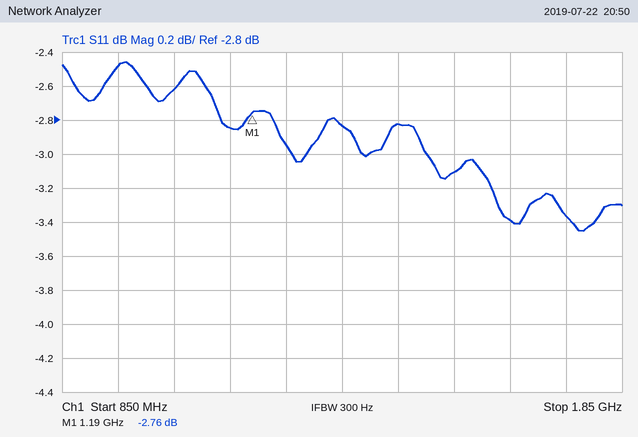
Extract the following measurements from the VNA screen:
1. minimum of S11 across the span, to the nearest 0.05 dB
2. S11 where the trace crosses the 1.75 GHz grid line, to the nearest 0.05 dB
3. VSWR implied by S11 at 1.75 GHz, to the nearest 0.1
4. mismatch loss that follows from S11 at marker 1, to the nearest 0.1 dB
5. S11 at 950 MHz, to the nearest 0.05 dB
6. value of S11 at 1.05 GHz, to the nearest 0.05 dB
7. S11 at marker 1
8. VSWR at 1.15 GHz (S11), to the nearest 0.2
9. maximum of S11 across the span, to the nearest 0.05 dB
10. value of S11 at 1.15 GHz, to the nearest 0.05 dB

-3.45 dB
-3.35 dB
5.2
3.3 dB
-2.50 dB
-2.60 dB
-2.76 dB
6.2
-2.45 dB
-2.85 dB
